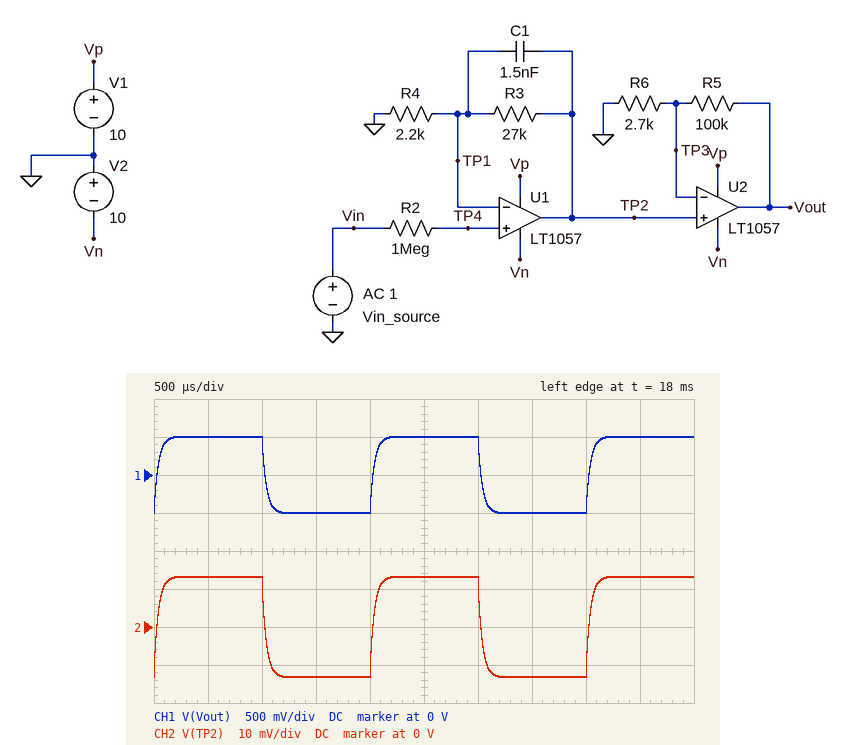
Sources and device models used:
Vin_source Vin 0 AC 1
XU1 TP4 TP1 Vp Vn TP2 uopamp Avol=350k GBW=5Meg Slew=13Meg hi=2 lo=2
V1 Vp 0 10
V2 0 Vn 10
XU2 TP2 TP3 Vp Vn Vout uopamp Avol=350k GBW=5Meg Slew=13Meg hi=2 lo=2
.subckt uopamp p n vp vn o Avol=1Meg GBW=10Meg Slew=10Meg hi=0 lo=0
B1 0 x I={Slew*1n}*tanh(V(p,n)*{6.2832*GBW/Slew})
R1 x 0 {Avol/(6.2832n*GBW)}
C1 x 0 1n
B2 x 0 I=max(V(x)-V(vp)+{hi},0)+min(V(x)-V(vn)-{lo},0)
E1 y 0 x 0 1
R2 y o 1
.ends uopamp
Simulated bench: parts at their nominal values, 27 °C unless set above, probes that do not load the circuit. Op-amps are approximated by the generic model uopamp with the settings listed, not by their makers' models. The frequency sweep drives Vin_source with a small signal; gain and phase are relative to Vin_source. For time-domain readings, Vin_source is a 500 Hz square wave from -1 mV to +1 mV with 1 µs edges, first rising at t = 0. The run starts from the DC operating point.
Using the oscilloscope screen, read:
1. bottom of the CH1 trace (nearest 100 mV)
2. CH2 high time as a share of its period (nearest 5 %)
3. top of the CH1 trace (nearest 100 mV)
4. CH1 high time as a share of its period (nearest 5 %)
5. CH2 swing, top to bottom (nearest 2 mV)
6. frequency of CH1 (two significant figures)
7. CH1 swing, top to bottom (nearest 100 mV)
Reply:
-500 mV
50 %
500 mV
50 %
26 mV
500 Hz
1.0 V
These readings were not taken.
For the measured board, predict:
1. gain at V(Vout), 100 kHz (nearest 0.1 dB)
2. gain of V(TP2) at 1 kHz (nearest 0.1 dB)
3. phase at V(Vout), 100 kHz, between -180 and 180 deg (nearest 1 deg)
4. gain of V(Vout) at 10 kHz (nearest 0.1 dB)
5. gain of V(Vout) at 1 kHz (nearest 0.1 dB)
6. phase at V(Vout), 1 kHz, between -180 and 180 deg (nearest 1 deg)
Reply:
30.6 dB
22.2 dB
-64 deg
45.4 dB
53.8 dB
-14 deg
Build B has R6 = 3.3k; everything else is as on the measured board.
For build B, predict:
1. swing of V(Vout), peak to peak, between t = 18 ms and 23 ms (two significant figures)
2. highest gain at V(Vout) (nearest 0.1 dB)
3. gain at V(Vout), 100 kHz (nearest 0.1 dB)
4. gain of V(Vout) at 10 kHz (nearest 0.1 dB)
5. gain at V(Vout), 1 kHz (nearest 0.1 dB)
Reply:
830 mV
52.4 dB
29.4 dB
43.7 dB
52.1 dB
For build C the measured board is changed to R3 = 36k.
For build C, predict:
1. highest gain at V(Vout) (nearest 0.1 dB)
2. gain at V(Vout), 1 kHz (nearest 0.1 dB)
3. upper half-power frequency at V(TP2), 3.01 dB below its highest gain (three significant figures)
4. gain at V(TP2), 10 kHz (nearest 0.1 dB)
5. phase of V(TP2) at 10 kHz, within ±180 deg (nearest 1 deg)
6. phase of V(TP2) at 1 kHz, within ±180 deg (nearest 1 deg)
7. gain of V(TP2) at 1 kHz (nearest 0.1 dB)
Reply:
56.4 dB
55.9 dB
2.93 kHz
13.9 dB
-63 deg
-18 deg
24.3 dB
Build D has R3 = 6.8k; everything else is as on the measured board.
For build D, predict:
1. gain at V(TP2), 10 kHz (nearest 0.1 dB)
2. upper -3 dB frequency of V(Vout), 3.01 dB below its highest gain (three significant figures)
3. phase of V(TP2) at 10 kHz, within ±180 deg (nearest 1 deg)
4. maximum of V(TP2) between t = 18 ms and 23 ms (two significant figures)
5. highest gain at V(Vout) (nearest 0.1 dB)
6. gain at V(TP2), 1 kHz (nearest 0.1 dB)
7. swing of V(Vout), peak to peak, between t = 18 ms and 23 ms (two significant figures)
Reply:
10.8 dB
16.2 kHz
-24 deg
4.1 mV
43.8 dB
12.2 dB
310 mV
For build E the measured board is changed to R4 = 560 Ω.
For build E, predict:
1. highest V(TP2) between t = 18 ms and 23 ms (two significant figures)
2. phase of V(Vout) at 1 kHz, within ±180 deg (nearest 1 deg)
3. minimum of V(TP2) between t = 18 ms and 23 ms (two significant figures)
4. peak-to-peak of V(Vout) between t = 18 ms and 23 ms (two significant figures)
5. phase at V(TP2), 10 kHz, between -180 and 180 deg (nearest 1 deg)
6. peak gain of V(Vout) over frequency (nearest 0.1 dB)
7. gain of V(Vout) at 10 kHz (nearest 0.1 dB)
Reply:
49 mV
-15 deg
-49 mV
3.7 V
-66 deg
65.4 dB
56.4 dB
